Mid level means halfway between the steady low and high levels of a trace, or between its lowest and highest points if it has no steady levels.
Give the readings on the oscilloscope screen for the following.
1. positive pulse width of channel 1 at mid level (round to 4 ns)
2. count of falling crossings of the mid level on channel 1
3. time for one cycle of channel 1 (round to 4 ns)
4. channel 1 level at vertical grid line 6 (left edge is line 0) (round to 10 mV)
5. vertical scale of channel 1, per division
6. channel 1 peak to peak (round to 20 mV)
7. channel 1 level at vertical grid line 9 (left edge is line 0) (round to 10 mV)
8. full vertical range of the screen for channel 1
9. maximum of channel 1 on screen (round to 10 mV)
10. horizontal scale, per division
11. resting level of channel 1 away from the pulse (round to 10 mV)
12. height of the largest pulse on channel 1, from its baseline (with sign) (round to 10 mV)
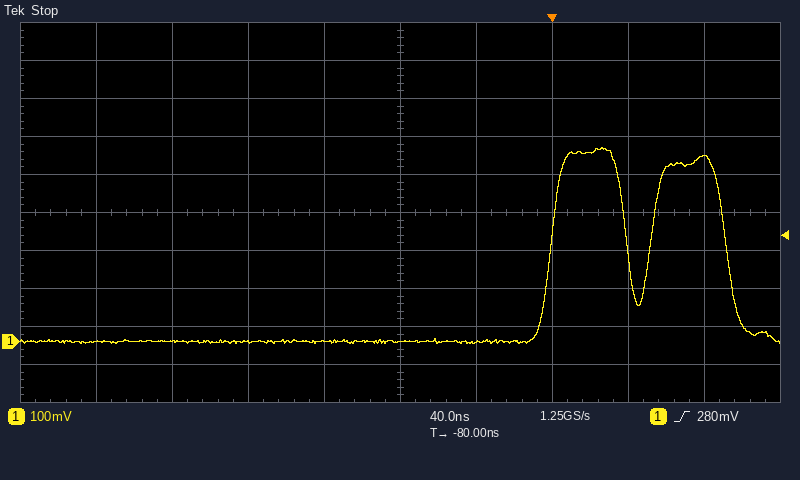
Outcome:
40 ns
2
52 ns
0 mV
100 mV
520 mV
490 mV
1 V
510 mV
40 ns
0 mV
+510 mV
